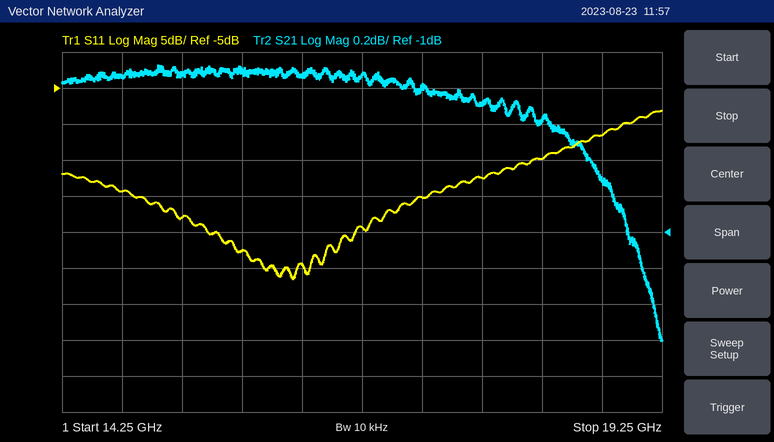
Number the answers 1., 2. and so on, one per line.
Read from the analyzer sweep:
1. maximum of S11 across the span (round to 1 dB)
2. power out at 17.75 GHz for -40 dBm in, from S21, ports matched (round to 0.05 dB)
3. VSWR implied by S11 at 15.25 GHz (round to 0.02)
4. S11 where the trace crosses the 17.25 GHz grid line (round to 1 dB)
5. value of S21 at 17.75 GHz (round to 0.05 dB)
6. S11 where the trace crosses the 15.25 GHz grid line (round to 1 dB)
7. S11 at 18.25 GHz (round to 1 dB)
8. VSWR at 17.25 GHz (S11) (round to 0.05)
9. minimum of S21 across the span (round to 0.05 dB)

1. -8 dB
2. -40.30 dBm
3. 1.16
4. -20 dB
5. -0.30 dB
6. -23 dB
7. -15 dB
8. 1.20
9. -1.60 dB
